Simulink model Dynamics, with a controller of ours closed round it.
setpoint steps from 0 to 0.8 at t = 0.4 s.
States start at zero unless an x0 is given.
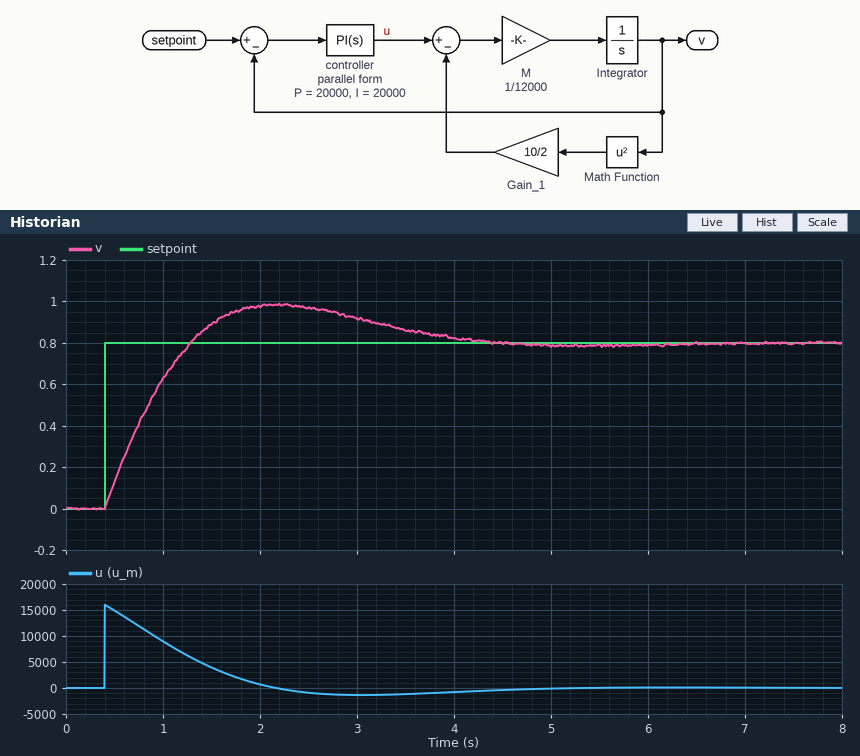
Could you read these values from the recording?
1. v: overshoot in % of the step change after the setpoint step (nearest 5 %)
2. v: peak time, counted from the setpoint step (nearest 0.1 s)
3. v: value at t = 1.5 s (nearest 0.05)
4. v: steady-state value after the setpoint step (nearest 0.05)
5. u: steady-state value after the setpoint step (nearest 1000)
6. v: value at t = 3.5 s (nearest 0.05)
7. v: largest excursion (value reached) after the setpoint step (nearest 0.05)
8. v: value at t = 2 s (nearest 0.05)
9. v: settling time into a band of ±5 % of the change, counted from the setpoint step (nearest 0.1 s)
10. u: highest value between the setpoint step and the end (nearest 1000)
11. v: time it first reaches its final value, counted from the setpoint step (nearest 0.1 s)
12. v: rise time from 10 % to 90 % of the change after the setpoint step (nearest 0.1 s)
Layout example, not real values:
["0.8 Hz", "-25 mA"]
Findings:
["25 %", "1.8 s", "0.90", "0.80", "0", "0.85", "1.00", "1.00", "3.4 s", "16000", "0.9 s", "0.7 s"]
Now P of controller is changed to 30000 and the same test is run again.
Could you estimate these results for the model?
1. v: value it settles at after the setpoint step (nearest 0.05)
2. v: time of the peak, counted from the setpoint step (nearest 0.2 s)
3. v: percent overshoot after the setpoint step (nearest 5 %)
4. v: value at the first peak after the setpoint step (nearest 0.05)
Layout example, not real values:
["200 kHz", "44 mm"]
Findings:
["0.80", "1.6 s", "15 %", "0.90"]
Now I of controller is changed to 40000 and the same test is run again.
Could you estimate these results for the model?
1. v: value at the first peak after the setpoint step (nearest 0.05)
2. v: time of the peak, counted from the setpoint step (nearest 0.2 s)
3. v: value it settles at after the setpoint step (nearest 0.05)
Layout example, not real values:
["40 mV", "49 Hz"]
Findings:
["1.05", "1.4 s", "0.80"]
